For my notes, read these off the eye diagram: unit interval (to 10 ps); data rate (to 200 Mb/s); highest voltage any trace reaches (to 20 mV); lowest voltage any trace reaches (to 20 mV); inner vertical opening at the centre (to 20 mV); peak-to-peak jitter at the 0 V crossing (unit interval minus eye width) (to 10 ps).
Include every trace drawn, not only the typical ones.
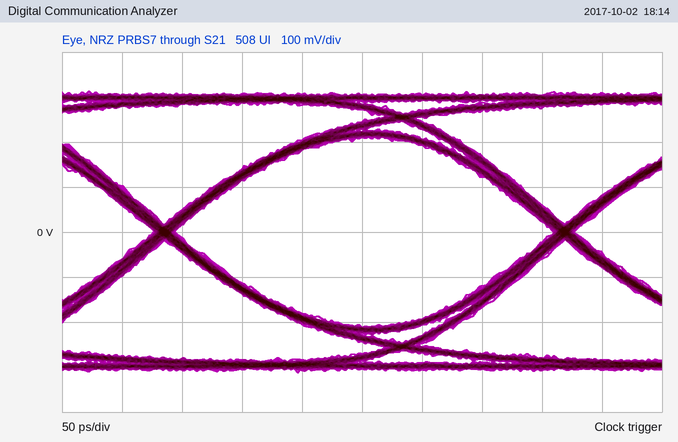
330 ps
3.0 Gb/s
320 mV
-320 mV
420 mV
20 ps
